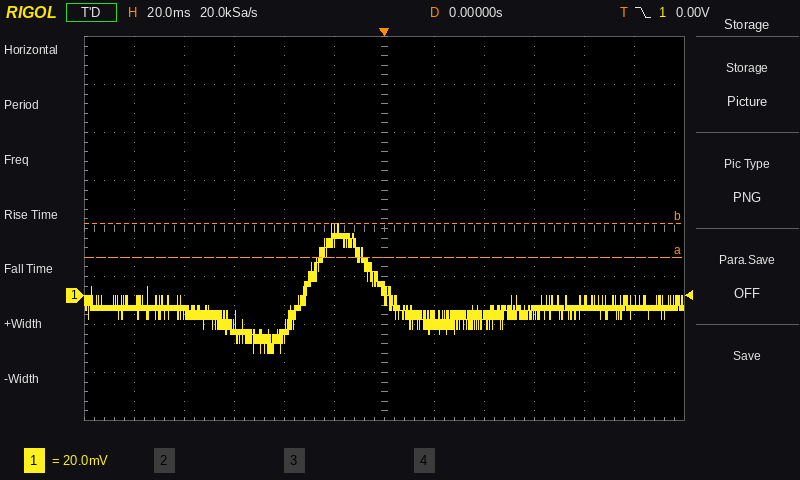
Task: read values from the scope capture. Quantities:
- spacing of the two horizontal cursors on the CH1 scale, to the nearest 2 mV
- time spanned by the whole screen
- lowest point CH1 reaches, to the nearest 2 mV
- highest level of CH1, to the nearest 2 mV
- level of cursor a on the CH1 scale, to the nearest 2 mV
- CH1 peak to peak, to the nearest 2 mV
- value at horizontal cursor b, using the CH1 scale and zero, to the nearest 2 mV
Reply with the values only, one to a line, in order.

14 mV
240 ms
-24 mV
30 mV
16 mV
54 mV
30 mV
